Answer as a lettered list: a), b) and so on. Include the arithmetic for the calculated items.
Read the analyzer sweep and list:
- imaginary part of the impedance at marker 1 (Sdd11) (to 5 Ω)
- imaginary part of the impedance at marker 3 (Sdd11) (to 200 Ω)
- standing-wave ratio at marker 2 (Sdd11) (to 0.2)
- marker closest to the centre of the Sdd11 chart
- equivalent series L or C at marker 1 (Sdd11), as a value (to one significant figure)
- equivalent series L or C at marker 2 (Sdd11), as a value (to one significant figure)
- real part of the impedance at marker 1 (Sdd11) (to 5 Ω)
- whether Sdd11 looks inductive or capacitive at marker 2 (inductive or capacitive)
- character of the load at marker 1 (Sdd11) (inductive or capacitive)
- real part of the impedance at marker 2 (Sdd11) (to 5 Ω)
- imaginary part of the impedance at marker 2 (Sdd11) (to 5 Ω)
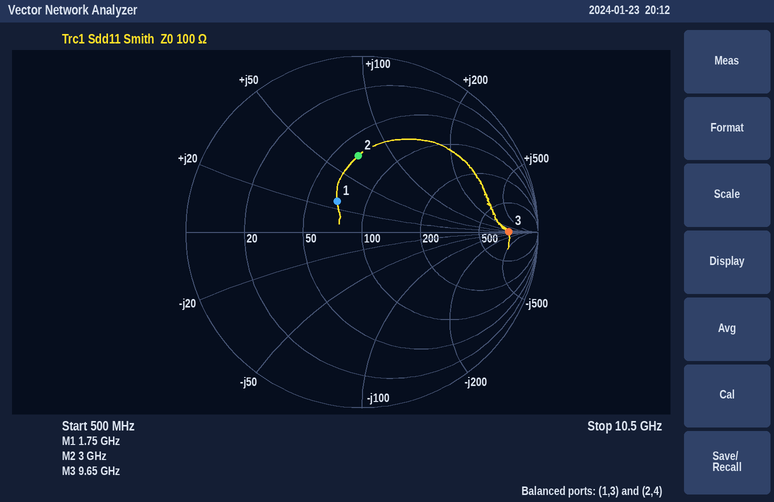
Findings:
a) +25 Ω
b) 0 Ω
c) 2.6
d) marker 1
e) L = 25 Ω/(2π × 1.75 GHz) ≈ 2 nH
f) L = 70 Ω/(2π × 3 GHz) ≈ 4 nH
g) 70 Ω
h) inductive
i) inductive
j) 65 Ω
k) +70 Ω
